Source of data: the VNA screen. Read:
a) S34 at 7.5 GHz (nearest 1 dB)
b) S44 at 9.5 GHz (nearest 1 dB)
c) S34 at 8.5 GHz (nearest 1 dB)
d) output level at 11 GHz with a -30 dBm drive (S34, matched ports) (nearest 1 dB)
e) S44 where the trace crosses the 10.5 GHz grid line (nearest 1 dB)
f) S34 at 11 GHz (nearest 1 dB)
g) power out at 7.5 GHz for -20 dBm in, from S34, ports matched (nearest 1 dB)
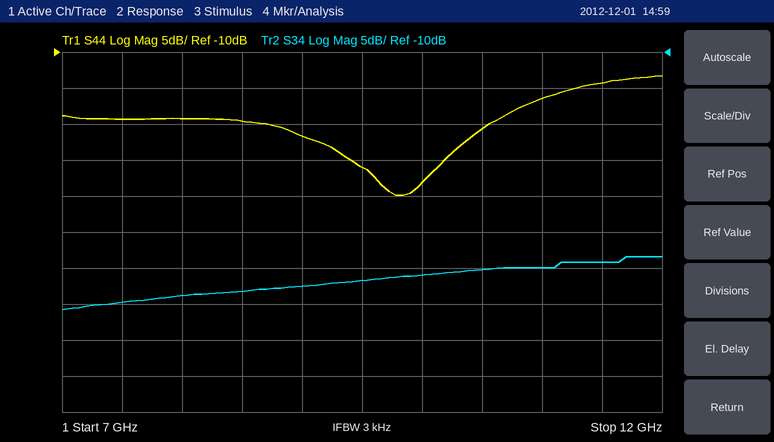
-45 dB
-26 dB
-43 dB
-70 dBm
-21 dB
-40 dB
-65 dBm
